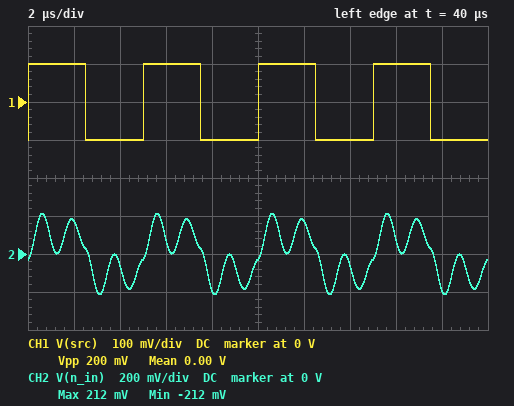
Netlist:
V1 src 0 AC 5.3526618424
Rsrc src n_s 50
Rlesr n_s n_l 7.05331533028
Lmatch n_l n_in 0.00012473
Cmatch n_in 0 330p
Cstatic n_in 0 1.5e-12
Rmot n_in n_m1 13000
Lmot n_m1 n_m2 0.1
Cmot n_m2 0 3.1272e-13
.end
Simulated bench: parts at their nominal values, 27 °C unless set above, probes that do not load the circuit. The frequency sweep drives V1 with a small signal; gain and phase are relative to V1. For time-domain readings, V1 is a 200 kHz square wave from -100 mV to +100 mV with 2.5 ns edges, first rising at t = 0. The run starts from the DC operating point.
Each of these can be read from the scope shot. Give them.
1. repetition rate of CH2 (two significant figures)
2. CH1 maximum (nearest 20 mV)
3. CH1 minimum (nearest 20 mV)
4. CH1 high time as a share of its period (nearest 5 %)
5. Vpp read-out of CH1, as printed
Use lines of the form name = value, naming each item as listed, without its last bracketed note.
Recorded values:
repetition rate of CH2 = 200 kHz
CH1 maximum = 100 mV
CH1 minimum = -100 mV
CH1 high time as a share of its period = 50 %
Vpp read-out of CH1, as printed = 200 mV
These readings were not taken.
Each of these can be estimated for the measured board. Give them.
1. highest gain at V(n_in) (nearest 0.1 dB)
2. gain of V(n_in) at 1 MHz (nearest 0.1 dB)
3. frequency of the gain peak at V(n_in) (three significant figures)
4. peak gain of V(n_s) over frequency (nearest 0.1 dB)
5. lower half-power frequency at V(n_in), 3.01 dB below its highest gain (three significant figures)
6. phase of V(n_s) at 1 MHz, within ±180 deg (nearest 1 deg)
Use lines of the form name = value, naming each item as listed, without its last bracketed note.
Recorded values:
highest gain at V(n_in) = 20.6 dB
gain of V(n_in) at 1 MHz = 3.9 dB
frequency of the gain peak at V(n_in) = 779 kHz
peak gain of V(n_s) over frequency = 0 dB
lower half-power frequency at V(n_in), 3.01 dB below its highest gain = 742 kHz
phase of V(n_s) at 1 MHz, within ±180 deg = 9 deg
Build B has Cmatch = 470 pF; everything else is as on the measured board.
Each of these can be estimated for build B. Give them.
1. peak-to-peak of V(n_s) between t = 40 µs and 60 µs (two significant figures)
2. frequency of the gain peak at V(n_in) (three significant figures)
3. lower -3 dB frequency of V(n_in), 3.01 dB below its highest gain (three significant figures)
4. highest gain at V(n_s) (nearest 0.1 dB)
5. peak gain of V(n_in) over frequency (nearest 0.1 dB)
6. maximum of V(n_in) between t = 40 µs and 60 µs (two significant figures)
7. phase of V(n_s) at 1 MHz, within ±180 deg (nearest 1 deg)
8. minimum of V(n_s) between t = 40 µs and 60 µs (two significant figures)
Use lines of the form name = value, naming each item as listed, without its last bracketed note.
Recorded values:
peak-to-peak of V(n_s) between t = 40 µs and 60 µs = 240 mV
frequency of the gain peak at V(n_in) = 654 kHz
lower -3 dB frequency of V(n_in), 3.01 dB below its highest gain = 616 kHz
highest gain at V(n_s) = 0 dB
peak gain of V(n_in) over frequency = 19.1 dB
maximum of V(n_in) between t = 40 µs and 60 µs = 330 mV
phase of V(n_s) at 1 MHz, within ±180 deg = 6 deg
minimum of V(n_s) between t = 40 µs and 60 µs = -120 mV
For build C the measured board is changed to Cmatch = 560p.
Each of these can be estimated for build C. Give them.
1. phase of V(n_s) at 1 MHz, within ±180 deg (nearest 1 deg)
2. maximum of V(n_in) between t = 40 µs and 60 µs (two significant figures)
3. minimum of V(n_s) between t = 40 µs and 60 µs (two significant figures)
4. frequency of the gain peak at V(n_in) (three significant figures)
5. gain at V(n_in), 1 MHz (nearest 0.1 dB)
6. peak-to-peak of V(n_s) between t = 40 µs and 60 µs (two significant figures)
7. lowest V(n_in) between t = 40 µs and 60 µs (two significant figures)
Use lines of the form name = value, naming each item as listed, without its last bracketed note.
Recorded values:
phase of V(n_s) at 1 MHz, within ±180 deg = 6 deg
maximum of V(n_in) between t = 40 µs and 60 µs = 480 mV
minimum of V(n_s) between t = 40 µs and 60 µs = -140 mV
frequency of the gain peak at V(n_in) = 599 kHz
gain at V(n_in), 1 MHz = -5.0 dB
peak-to-peak of V(n_s) between t = 40 µs and 60 µs = 270 mV
lowest V(n_in) between t = 40 µs and 60 µs = -480 mV
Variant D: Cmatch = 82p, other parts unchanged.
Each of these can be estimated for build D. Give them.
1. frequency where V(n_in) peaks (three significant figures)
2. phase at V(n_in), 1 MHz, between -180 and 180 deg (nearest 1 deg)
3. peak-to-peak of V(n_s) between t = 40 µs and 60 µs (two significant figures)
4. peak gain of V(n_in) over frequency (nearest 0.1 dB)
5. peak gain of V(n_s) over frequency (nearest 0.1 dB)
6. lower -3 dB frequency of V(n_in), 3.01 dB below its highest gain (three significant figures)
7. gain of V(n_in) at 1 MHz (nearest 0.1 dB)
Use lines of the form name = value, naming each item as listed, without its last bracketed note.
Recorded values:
frequency where V(n_in) peaks = 1.56 MHz
phase at V(n_in), 1 MHz, between -180 and 180 deg = -3 deg
peak-to-peak of V(n_s) between t = 40 µs and 60 µs = 210 mV
peak gain of V(n_in) over frequency = 26.6 dB
peak gain of V(n_s) over frequency = 0 dB
lower -3 dB frequency of V(n_in), 3.01 dB below its highest gain = 1.52 MHz
gain of V(n_in) at 1 MHz = 4.5 dB
